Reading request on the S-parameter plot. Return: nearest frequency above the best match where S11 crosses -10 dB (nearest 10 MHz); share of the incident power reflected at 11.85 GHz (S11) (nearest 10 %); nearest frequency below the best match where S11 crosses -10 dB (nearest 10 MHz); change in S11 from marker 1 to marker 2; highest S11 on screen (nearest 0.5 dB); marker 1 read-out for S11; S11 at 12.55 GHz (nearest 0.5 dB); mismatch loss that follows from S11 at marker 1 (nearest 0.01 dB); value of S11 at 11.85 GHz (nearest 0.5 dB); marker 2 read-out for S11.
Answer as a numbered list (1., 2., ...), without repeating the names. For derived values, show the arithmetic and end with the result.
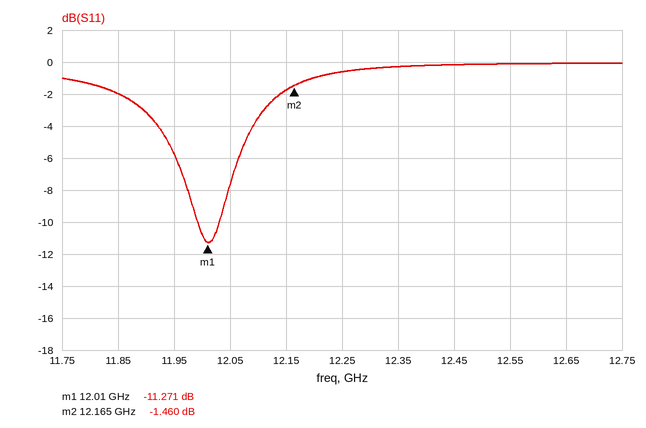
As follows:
1. 12.03 GHz
2. 10^(-2/10) ≈ 63.1 %, so 60 % to the nearest 10 %
3. 11.99 GHz
4. -1.46 − (-11.271) = 9.811 dB
5. 0.0 dB
6. -11.271 dB
7. 0.0 dB
8. −10 log10(1 − 10^(-11.271/10)) ≈ 0.34 dB
9. -2.0 dB
10. -1.460 dB
